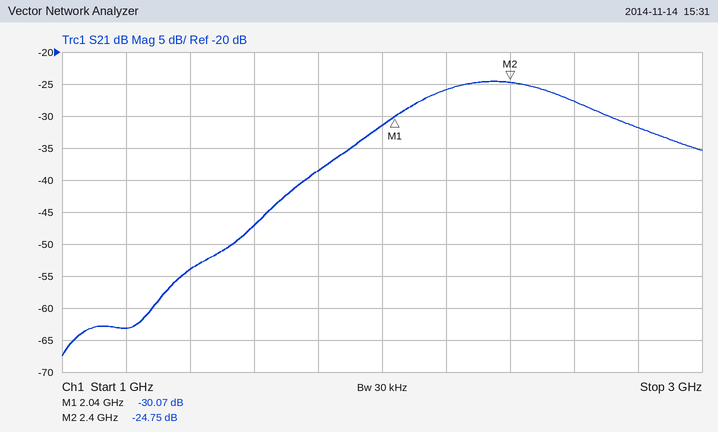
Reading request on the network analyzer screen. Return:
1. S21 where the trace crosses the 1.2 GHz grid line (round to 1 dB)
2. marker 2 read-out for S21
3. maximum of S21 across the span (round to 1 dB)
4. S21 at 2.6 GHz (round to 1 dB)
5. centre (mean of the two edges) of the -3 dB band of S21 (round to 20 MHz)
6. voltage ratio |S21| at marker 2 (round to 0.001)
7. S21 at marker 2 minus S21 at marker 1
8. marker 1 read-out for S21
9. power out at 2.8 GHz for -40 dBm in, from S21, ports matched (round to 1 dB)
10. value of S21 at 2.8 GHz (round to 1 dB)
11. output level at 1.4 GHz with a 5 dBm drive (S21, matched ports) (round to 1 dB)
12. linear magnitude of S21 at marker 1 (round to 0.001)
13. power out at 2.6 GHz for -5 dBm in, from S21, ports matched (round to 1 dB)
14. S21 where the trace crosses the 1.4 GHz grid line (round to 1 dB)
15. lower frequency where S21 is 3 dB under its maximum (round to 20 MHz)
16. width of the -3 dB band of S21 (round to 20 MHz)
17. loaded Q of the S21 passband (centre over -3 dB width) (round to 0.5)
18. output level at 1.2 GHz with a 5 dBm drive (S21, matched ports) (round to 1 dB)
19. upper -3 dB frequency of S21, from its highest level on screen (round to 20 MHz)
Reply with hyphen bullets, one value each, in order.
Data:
- -63 dB
- -24.75 dB
- -25 dB
- -28 dB
- 2.36 GHz
- 0.058
- 5.32 dB
- -30.07 dB
- -72 dBm
- -32 dB
- -49 dBm
- 0.031
- -33 dBm
- -54 dB
- 2.12 GHz
- 480 MHz
- 5.0
- -58 dBm
- 2.60 GHz
